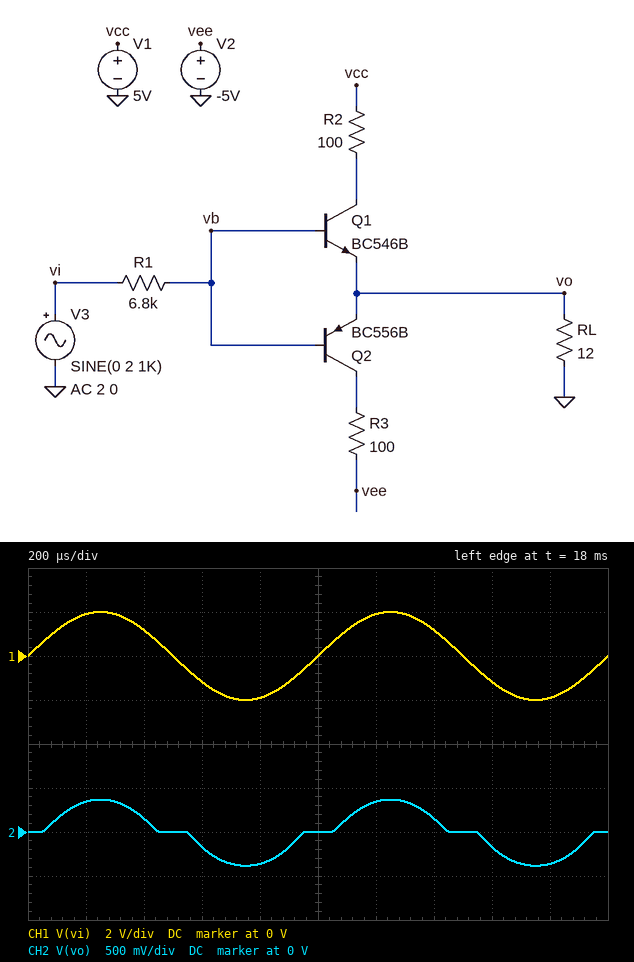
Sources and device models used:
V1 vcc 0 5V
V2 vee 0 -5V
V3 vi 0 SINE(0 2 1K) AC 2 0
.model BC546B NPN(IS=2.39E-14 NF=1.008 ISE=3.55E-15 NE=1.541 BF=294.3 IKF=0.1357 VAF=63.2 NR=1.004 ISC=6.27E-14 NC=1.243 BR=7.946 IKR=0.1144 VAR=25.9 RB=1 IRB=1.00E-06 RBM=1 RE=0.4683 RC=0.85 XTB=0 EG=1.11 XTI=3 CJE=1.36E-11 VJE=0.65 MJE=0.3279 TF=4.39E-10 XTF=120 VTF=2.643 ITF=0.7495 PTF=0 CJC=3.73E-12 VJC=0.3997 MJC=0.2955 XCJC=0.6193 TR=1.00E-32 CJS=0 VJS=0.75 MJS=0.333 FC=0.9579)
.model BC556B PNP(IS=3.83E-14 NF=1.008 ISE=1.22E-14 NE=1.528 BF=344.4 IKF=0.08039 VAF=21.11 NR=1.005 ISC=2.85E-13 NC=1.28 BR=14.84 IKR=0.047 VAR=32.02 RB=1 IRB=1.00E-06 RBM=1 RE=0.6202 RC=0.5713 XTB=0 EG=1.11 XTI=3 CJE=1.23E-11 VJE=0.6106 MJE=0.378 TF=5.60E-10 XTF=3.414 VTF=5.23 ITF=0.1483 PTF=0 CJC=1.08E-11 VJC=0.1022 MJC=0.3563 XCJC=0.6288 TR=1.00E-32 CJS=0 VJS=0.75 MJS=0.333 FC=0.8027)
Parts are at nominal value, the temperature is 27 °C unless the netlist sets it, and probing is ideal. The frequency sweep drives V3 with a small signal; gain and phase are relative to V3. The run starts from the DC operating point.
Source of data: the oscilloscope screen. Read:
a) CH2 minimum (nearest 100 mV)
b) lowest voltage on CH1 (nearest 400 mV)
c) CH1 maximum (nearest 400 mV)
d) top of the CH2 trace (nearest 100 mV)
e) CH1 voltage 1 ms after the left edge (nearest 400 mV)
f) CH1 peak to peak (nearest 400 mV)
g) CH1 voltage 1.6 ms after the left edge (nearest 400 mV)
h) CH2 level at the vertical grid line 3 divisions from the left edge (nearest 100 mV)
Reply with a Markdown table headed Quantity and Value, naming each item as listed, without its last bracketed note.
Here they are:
| Quantity | Value |
|---|---|
| CH2 minimum | -400 mV |
| lowest voltage on CH1 | -2.0 V |
| CH1 maximum | 2.0 V |
| top of the CH2 trace | 400 mV |
| CH1 voltage 1 ms after the left edge | 0 V |
| CH1 peak to peak | 4.0 V |
| CH1 voltage 1.6 ms after the left edge | -1.2 V |
| CH2 level at the vertical grid line 3 divisions from the left edge | -200 mV |
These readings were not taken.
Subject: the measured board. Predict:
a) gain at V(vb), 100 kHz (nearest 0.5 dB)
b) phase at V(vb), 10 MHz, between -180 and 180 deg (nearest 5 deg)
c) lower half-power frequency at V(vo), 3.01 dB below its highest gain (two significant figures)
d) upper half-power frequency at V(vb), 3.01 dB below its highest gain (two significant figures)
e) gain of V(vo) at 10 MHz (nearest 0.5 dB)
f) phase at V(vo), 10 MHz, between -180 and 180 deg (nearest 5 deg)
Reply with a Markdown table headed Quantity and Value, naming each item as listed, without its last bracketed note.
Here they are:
| Quantity | Value |
|---|---|
| gain at V(vb), 100 kHz | 0 dB |
| phase at V(vb), 10 MHz, between -180 and 180 deg | -85 deg |
| lower half-power frequency at V(vo), 3.01 dB below its highest gain | 770 kHz |
| upper half-power frequency at V(vb), 3.01 dB below its highest gain | 770 kHz |
| gain of V(vo) at 10 MHz | -56.5 dB |
| phase at V(vo), 10 MHz, between -180 and 180 deg | 5 deg |
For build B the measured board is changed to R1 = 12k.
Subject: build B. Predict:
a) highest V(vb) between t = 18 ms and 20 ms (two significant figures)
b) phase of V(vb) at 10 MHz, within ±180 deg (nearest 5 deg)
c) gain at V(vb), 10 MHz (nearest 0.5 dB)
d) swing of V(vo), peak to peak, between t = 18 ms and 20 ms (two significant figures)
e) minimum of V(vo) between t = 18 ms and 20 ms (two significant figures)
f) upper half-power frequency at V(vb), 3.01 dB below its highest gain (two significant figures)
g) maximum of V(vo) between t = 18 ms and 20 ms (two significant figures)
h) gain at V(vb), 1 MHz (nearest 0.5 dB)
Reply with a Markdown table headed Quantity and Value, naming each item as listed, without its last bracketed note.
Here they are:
| Quantity | Value |
|---|---|
| highest V(vb) between t = 18 ms and 20 ms | 990 mV |
| phase of V(vb) at 10 MHz, within ±180 deg | -85 deg |
| gain at V(vb), 10 MHz | -27.0 dB |
| swing of V(vo), peak to peak, between t = 18 ms and 20 ms | 540 mV |
| minimum of V(vo) between t = 18 ms and 20 ms | -280 mV |
| upper half-power frequency at V(vb), 3.01 dB below its highest gain | 440 kHz |
| maximum of V(vo) between t = 18 ms and 20 ms | 260 mV |
| gain at V(vb), 1 MHz | -8.0 dB |
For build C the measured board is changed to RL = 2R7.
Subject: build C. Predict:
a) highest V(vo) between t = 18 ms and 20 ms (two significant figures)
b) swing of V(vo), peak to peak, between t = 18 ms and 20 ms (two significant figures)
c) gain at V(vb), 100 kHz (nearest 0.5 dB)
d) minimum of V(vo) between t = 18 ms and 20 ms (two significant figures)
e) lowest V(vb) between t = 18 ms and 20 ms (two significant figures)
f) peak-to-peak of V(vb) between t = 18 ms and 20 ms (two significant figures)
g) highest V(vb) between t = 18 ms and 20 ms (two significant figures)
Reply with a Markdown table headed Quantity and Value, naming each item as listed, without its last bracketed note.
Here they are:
| Quantity | Value |
|---|---|
| highest V(vo) between t = 18 ms and 20 ms | 100 mV |
| swing of V(vo), peak to peak, between t = 18 ms and 20 ms | 210 mV |
| gain at V(vb), 100 kHz | 0 dB |
| minimum of V(vo) between t = 18 ms and 20 ms | -100 mV |
| lowest V(vb) between t = 18 ms and 20 ms | -860 mV |
| peak-to-peak of V(vb) between t = 18 ms and 20 ms | 1.7 V |
| highest V(vb) between t = 18 ms and 20 ms | 860 mV |
